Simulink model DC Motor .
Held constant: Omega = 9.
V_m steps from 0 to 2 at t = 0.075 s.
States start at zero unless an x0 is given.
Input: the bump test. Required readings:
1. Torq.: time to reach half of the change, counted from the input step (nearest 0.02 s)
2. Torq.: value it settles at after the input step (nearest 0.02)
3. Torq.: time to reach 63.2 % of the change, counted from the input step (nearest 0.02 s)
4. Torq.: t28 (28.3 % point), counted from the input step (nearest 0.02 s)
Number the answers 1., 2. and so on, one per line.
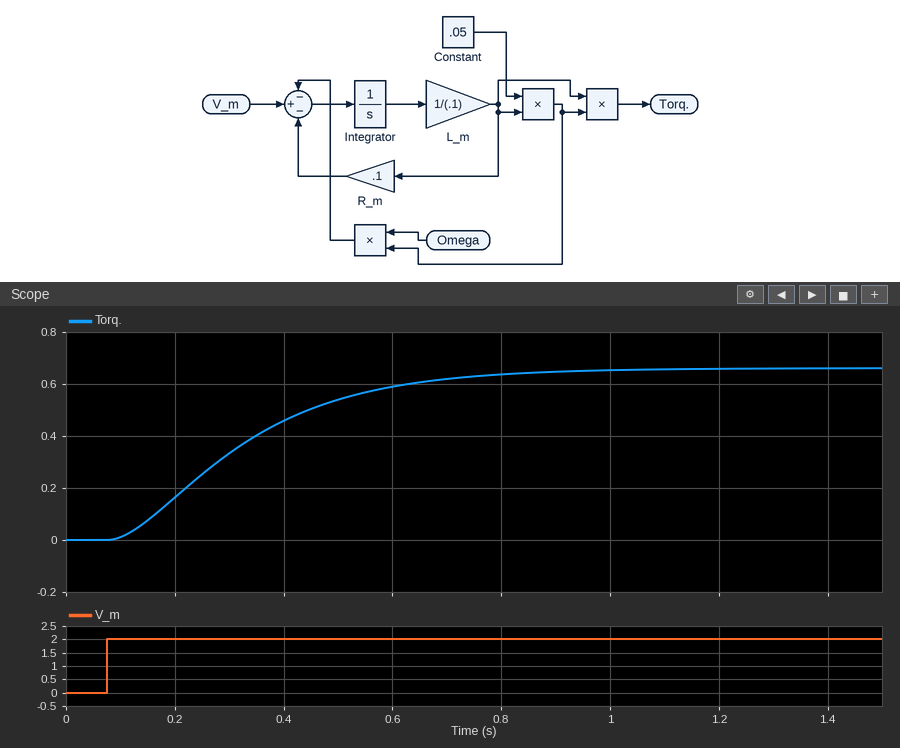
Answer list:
1. 0.22 s
2. 0.66
3. 0.28 s
4. 0.14 s
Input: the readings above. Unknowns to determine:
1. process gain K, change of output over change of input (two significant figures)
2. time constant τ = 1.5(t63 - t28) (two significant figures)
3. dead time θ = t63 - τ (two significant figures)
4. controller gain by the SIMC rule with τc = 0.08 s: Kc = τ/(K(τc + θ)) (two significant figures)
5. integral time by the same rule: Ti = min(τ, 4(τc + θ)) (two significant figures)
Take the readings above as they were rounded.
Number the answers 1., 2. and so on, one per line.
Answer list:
1. 0.33
2. 0.21 s
3. 0.070 s
4. 4.2
5. 0.21 s
